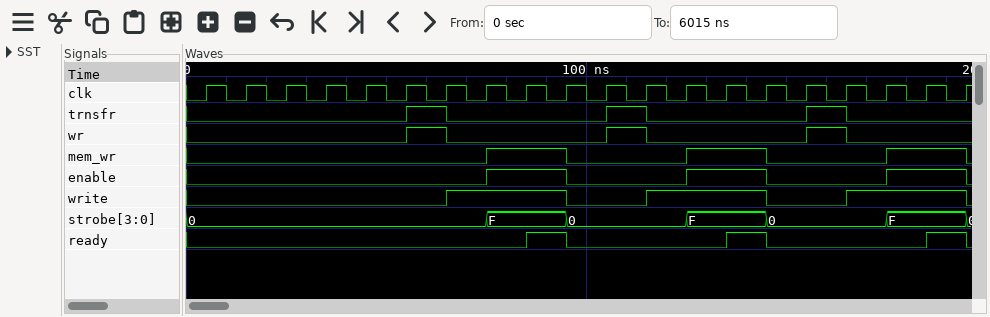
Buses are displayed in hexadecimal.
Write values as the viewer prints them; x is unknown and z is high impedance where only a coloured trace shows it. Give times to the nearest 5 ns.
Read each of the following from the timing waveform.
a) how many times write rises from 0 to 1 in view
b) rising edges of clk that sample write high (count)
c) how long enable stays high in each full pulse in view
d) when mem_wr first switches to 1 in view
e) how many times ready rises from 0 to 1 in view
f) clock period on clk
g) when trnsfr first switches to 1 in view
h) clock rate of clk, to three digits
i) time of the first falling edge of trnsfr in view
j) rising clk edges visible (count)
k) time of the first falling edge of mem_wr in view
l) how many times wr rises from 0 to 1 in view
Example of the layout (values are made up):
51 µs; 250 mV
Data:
3; 9; 20 ns, 20 ns, 20 ns; 75 ns; 3; 10 ns; 55 ns; 100 MHz; 65 ns; 20; 95 ns; 3
